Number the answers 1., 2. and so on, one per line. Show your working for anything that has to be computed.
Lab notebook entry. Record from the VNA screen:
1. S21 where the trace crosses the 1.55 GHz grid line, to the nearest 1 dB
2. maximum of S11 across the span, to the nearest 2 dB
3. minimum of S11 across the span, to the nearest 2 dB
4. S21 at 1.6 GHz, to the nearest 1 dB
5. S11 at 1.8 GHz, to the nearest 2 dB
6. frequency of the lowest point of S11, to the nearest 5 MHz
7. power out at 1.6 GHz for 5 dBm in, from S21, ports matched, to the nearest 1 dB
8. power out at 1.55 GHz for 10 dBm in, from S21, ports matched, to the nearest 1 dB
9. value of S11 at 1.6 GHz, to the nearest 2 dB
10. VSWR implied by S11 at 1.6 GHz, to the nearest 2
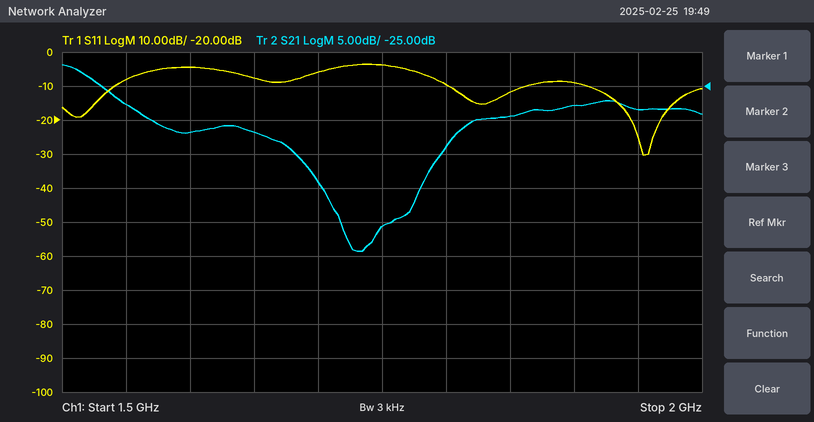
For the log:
1. -28 dB
2. -4 dB
3. -30 dB
4. -32 dB
5. -10 dB
6. 1.955 GHz
7. 5 dBm + (-32 dB) = -27 dBm
8. 10 dBm + (-28 dB) = -18 dBm
9. -4 dB
10. |Γ| = 10^(-4/20) = 0.6310; VSWR = (1 + 0.6310)/(1 − 0.6310) ≈ 4
